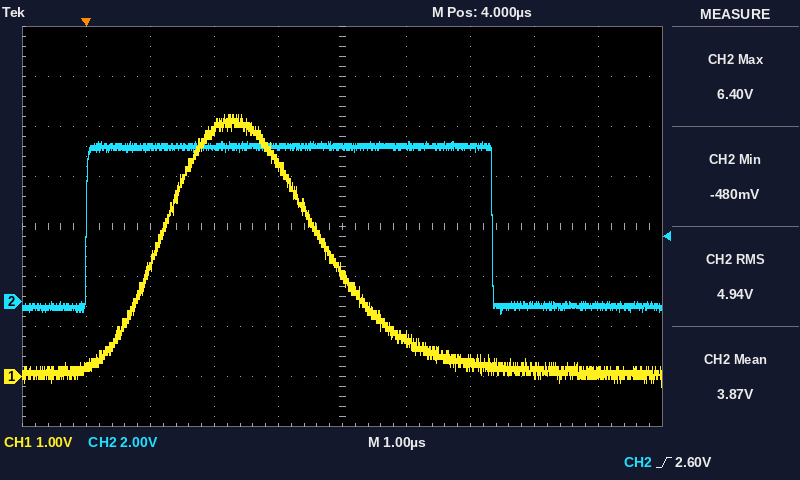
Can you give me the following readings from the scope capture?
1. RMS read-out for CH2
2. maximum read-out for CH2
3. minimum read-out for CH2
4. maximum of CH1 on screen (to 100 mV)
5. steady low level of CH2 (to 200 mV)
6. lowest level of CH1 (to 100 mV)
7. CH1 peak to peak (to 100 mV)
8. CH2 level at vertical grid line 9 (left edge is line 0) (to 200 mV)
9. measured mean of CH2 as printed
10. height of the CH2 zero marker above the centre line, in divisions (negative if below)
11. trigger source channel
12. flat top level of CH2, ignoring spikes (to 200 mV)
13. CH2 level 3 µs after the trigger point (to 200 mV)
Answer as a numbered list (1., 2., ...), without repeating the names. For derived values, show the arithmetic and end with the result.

1. 4.94 V
2. 6.40 V
3. -480 mV
4. 5.2 V
5. -200 mV
6. -200 mV
7. 5.2 V − (-200 mV) = 5.4 V
8. -200 mV
9. 3.87 V
10. -1.5 div
11. CH2
12. 6.2 V
13. 6.2 V
